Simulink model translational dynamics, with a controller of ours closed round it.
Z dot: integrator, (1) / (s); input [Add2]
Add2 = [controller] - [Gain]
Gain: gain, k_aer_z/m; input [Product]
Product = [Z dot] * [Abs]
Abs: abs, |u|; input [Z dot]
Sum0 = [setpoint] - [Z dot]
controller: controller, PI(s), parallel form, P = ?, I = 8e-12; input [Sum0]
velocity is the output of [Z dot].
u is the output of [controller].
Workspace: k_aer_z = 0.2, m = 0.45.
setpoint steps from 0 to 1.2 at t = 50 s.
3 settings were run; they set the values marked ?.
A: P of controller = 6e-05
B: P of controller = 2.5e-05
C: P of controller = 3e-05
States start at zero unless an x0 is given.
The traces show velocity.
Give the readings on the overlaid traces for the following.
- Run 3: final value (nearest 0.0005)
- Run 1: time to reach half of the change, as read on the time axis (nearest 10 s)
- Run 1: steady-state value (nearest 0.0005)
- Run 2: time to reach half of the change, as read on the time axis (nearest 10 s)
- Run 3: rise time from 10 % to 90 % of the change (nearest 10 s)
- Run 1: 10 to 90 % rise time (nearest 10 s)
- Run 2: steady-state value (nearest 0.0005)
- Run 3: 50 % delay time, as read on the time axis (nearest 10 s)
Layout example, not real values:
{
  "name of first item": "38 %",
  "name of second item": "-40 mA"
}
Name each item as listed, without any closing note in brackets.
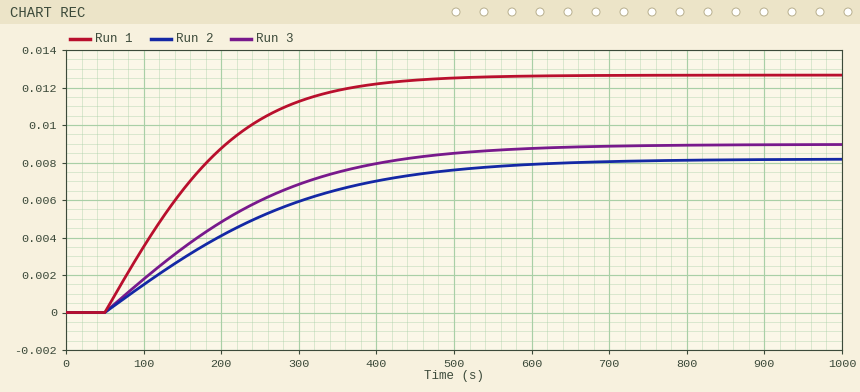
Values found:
{
  "Run 3: final value": "0.0090",
  "Run 1: time to reach half of the change, as read on the time axis": "150 s",
  "Run 1: steady-state value": "0.0125",
  "Run 2: time to reach half of the change, as read on the time axis": "200 s",
  "Run 3: rise time from 10 % to 90 % of the change": "340 s",
  "Run 1: 10 to 90 % rise time": "240 s",
  "Run 2: steady-state value": "0.0080",
  "Run 3: 50 % delay time, as read on the time axis": "190 s"
}
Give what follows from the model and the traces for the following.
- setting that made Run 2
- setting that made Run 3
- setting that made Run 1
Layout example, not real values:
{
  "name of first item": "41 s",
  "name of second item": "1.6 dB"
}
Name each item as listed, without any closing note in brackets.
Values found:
{
  "setting that made Run 2": "B",
  "setting that made Run 3": "C",
  "setting that made Run 1": "A"
}
